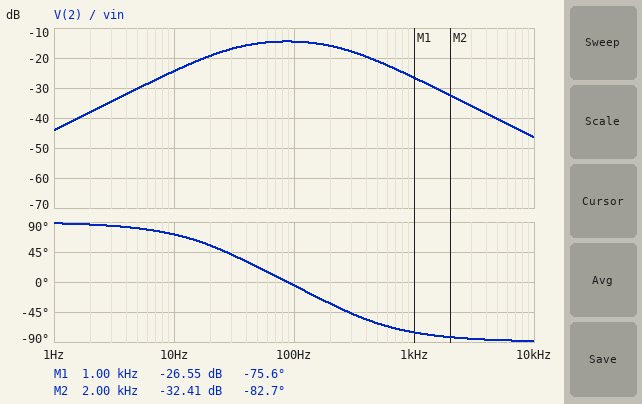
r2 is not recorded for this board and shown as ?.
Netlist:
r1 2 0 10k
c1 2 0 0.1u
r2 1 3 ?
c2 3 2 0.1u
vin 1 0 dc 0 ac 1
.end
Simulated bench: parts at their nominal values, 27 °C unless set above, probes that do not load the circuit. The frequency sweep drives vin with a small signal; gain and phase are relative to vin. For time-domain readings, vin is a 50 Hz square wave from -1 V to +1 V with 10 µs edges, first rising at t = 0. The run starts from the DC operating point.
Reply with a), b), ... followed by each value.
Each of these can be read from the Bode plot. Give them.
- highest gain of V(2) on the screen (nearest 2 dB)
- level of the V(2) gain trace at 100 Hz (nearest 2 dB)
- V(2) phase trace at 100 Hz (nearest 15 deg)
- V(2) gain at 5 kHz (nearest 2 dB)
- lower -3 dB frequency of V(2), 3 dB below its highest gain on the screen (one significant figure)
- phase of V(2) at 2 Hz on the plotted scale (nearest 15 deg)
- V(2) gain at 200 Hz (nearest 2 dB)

a) -14 dB
b) -14 dB
c) 0 deg
d) -40 dB
e) 30 Hz
f) 90 deg
g) -16 dB
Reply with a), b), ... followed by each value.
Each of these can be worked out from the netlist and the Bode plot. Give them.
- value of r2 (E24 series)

a) 33 kΩ
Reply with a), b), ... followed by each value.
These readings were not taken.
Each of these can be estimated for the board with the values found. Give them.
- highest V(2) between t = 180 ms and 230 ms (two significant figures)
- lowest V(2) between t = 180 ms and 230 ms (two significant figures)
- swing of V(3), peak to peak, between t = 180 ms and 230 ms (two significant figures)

a) 270 mV
b) -270 mV
c) 1.7 V
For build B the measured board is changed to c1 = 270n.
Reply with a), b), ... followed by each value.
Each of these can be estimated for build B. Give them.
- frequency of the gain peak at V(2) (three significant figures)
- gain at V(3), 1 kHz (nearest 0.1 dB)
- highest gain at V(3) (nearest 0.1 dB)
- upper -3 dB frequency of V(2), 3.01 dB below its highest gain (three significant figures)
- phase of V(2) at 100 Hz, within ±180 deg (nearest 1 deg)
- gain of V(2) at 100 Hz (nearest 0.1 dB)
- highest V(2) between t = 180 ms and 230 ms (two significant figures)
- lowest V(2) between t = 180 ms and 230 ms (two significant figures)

a) 53.3 Hz
b) -23.6 dB
c) 0 dB
d) 145 Hz
e) -30 deg
f) -18.1 dB
g) 180 mV
h) -180 mV
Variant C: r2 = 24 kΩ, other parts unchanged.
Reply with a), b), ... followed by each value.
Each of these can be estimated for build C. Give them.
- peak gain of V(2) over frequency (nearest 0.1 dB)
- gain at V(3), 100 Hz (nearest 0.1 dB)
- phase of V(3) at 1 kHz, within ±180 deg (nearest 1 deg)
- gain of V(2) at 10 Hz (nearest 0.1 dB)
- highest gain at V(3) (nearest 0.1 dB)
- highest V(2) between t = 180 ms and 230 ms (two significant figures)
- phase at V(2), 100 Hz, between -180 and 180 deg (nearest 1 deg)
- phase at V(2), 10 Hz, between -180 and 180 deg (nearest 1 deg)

a) -12.9 dB
b) -4.7 dB
c) -78 deg
d) -24.3 dB
e) 0 dB
f) 340 mV
g) 1 deg
h) 74 deg
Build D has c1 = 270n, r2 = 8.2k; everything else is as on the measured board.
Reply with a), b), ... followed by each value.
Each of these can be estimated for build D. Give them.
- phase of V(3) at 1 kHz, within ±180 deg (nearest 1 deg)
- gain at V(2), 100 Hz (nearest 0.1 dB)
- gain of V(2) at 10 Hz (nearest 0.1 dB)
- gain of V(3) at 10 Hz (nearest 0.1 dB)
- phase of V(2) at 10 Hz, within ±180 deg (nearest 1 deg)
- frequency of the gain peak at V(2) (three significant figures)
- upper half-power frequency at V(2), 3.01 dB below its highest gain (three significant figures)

a) -74 deg
b) -13.1 dB
c) -24.3 dB
d) 0 dB
e) 74 deg
f) 107 Hz
g) 357 Hz
